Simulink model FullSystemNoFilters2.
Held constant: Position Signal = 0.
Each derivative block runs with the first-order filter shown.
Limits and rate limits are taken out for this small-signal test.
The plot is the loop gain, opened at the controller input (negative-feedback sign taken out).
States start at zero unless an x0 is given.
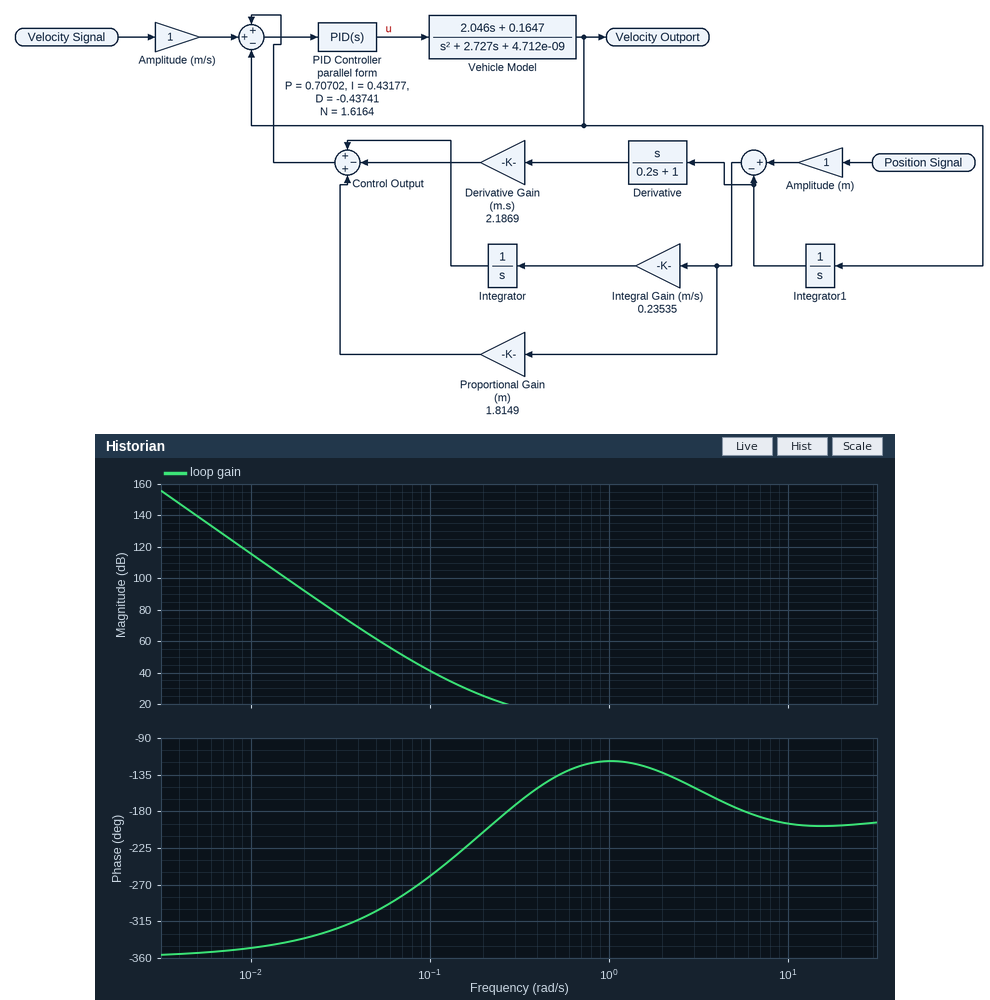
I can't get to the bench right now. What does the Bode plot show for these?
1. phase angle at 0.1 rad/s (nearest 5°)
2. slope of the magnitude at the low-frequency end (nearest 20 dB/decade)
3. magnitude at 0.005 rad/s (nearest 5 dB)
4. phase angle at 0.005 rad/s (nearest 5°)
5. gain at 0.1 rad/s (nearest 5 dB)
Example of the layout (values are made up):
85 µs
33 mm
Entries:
-260°
-80 dB/decade
140 dB
-355°
40 dB
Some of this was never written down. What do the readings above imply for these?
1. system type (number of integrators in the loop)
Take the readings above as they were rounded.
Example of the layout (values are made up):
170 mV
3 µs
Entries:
4
